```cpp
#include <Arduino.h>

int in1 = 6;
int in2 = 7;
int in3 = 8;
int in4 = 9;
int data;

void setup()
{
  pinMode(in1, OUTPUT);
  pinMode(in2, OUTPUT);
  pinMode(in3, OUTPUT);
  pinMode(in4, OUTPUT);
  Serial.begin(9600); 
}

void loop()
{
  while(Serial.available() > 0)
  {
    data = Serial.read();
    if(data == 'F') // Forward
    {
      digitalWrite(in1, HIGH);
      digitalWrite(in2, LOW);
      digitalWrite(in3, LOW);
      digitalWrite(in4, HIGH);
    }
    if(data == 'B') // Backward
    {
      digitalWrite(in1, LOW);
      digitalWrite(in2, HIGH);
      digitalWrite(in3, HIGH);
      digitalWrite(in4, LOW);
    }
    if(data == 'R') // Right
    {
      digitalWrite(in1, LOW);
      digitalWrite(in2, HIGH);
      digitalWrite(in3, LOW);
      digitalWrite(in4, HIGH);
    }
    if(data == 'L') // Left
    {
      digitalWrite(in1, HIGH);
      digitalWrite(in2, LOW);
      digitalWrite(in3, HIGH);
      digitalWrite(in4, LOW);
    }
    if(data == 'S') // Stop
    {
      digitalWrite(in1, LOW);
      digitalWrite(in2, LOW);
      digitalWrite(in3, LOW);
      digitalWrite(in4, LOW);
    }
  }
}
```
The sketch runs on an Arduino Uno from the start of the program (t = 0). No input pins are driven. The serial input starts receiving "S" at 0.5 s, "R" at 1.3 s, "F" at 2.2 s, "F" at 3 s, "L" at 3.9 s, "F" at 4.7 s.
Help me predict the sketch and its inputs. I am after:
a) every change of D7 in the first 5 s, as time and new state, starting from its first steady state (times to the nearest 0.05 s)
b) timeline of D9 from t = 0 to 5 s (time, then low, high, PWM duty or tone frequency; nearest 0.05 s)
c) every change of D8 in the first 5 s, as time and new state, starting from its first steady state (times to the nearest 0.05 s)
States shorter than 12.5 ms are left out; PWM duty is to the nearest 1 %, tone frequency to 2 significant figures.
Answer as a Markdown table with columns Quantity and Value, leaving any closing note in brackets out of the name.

| Quantity | Value |
|---|---|
| every change of D7 in the first 5 s, as time and new state, starting from its first steady state | 0 s low; 1.3 s high; 2.2 s low |
| timeline of D9 from t = 0 to 5 s | 0 s low; 1.3 s high; 3.9 s low; 4.7 s high |
| every change of D8 in the first 5 s, as time and new state, starting from its first steady state | 0 s low; 3.9 s high; 4.7 s low |
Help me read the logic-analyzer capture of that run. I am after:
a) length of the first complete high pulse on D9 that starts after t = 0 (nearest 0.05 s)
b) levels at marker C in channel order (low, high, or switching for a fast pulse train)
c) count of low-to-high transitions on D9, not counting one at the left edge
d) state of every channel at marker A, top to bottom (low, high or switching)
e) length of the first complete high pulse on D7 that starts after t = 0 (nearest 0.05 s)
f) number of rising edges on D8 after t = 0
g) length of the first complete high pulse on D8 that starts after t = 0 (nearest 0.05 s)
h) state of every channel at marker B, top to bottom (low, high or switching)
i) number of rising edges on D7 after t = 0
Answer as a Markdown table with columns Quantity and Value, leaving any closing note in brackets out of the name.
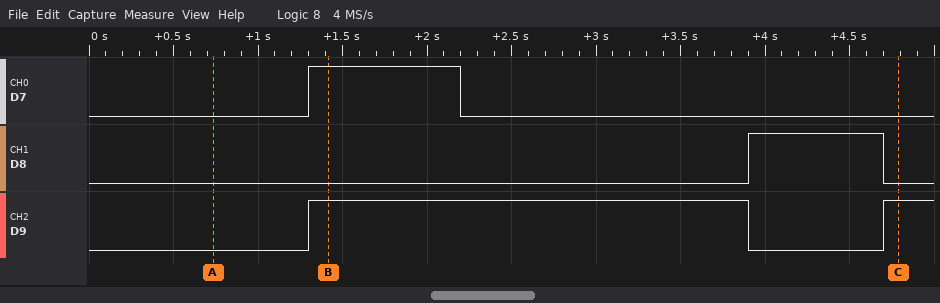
| Quantity | Value |
|---|---|
| length of the first complete high pulse on D9 that starts after t = 0 | 2.60 s |
| levels at marker C in channel order | D7 low, D8 low, D9 high |
| count of low-to-high transitions on D9, not counting one at the left edge | 2 |
| state of every channel at marker A, top to bottom | D7 low, D8 low, D9 low |
| length of the first complete high pulse on D7 that starts after t = 0 | 0.90 s |
| number of rising edges on D8 after t = 0 | 1 |
| length of the first complete high pulse on D8 that starts after t = 0 | 0.80 s |
| state of every channel at marker B, top to bottom | D7 high, D8 low, D9 high |
| number of rising edges on D7 after t = 0 | 1 |
